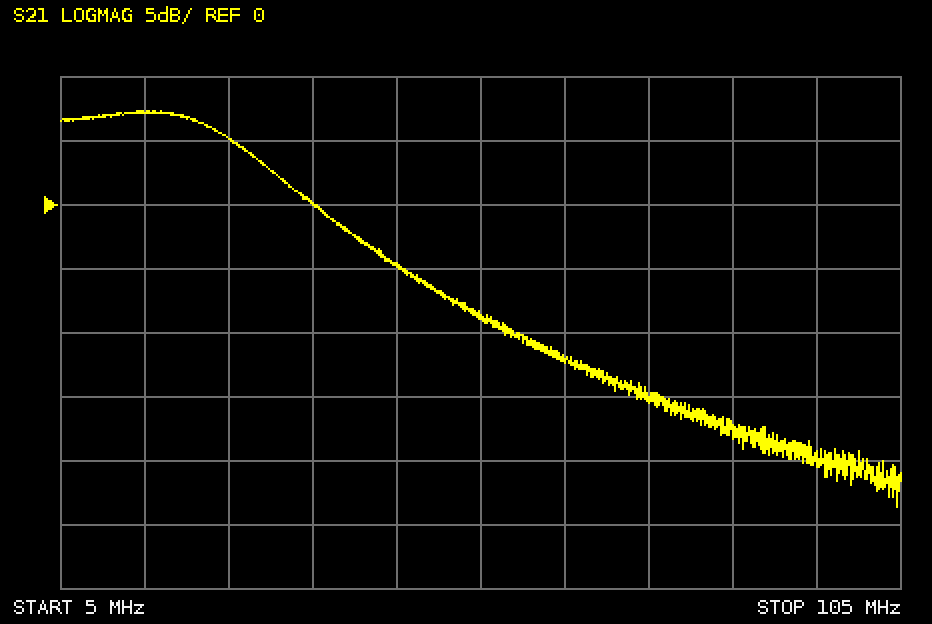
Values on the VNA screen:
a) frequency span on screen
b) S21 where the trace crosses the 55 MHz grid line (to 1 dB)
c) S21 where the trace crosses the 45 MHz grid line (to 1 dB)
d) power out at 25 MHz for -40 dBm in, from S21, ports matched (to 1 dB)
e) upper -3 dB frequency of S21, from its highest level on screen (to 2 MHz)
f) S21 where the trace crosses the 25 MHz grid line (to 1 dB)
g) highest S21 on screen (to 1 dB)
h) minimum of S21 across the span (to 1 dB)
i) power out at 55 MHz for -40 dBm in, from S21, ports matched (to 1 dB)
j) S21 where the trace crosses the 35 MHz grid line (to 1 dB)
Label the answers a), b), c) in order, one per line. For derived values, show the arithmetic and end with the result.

a) 100 MHz
b) -9 dB
c) -5 dB
d) -40 dBm + (5 dB) = -35 dBm
e) 26 MHz
f) 5 dB
g) 7 dB
h) -24 dB
i) -40 dBm + (-9 dB) = -49 dBm
j) 0 dB
